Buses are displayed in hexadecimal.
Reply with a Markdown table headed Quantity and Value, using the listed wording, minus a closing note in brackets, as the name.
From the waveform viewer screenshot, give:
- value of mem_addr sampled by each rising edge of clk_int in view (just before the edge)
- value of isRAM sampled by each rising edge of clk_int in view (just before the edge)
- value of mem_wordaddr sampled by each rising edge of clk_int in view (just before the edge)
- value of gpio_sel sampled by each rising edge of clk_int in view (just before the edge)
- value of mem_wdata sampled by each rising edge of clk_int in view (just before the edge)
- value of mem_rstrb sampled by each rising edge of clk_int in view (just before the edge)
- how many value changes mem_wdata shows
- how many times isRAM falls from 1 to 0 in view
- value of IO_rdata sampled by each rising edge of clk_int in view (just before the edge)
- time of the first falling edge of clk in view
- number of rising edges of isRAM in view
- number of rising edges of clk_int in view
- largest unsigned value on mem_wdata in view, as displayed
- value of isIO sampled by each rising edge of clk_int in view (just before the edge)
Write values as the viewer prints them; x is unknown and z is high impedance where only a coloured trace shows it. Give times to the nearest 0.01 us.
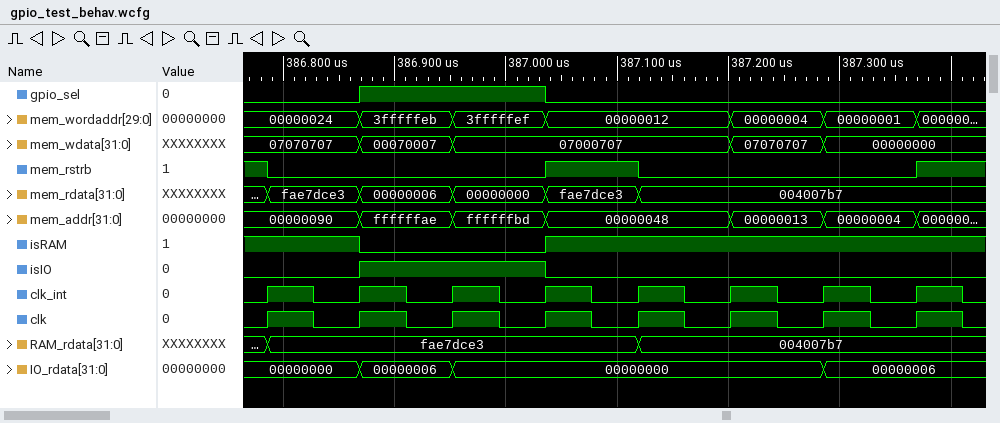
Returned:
| Quantity | Value |
|---|---|
| value of mem_addr sampled by each rising edge of clk_int in view | 00000090, 00000090, ffffffae, ffffffbd, 00000048, 00000048, 00000013, 00000004 |
| value of isRAM sampled by each rising edge of clk_int in view | 1 1 0 0 1 1 1 1 |
| value of mem_wordaddr sampled by each rising edge of clk_int in view | 00000024, 00000024, 3fffffeb, 3fffffef, 00000012, 00000012, 00000004, 00000001 |
| value of gpio_sel sampled by each rising edge of clk_int in view | 0 0 1 1 0 0 0 0 |
| value of mem_wdata sampled by each rising edge of clk_int in view | 07070707, 07070707, 00070007, 07000707, 07000707, 07000707, 07070707, 00000000 |
| value of mem_rstrb sampled by each rising edge of clk_int in view | 1 0 0 0 1 0 0 0 |
| how many value changes mem_wdata shows | 4 |
| how many times isRAM falls from 1 to 0 in view | 1 |
| value of IO_rdata sampled by each rising edge of clk_int in view | 00000000, 00000000, 00000006, 00000000, 00000000, 00000000, 00000000, 00000006 |
| time of the first falling edge of clk in view | 386.83 us |
| number of rising edges of isRAM in view | 1 |
| number of rising edges of clk_int in view | 8 |
| largest unsigned value on mem_wdata in view, as displayed | 07070707 |
| value of isIO sampled by each rising edge of clk_int in view | 0 0 1 1 0 0 0 0 |
